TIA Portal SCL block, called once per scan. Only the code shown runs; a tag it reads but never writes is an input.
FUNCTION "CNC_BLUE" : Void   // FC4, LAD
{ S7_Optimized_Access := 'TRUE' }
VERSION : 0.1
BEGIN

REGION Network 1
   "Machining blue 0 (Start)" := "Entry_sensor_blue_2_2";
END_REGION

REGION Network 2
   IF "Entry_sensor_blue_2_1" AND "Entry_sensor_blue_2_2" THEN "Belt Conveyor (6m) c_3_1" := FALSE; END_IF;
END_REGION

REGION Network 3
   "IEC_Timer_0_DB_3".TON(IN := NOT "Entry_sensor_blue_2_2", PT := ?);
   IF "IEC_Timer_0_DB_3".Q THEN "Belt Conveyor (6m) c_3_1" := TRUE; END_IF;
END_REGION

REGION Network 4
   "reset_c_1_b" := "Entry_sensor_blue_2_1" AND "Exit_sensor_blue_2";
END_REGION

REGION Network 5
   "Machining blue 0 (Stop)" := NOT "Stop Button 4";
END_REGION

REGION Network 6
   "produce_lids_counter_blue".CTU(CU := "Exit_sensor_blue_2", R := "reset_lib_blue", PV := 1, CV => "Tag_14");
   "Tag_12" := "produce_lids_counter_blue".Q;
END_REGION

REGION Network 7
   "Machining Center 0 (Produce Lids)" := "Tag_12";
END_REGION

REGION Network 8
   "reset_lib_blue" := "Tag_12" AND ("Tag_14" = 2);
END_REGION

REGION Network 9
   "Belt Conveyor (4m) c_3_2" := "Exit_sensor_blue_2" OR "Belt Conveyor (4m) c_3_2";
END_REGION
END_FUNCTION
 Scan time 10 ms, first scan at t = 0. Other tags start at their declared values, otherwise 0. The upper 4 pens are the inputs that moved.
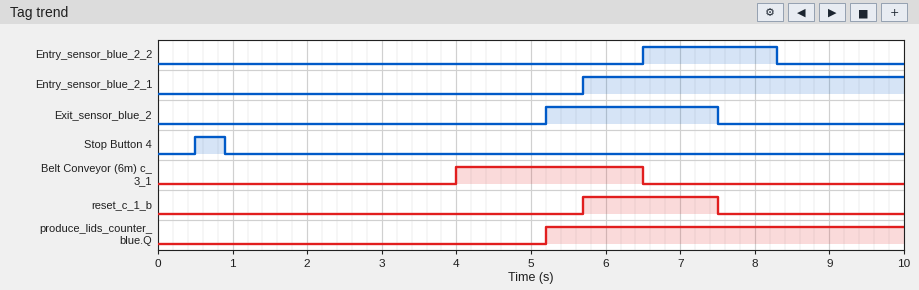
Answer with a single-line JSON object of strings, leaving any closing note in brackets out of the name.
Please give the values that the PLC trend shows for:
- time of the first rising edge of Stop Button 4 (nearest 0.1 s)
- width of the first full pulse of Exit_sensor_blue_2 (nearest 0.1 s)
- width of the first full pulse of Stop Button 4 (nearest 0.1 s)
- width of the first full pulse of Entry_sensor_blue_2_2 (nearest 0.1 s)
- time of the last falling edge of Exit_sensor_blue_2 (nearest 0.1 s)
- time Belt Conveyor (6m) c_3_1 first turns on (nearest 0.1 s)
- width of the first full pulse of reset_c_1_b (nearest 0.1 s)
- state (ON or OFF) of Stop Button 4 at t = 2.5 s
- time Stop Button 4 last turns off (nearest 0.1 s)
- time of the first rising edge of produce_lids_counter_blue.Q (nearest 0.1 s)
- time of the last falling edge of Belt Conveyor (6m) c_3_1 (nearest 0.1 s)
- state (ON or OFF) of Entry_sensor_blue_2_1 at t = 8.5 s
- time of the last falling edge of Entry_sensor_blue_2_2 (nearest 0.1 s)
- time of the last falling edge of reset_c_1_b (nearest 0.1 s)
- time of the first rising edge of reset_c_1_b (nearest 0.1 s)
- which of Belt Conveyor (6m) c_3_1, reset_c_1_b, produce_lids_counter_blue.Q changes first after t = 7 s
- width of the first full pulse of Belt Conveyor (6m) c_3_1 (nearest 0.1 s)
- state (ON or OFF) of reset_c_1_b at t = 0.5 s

{"time of the first rising edge of Stop Button 4": "0.5 s", "width of the first full pulse of Exit_sensor_blue_2": "2.3 s", "width of the first full pulse of Stop Button 4": "0.4 s", "width of the first full pulse of Entry_sensor_blue_2_2": "1.8 s", "time of the last falling edge of Exit_sensor_blue_2": "7.5 s", "time Belt Conveyor (6m) c_3_1 first turns on": "4.0 s", "width of the first full pulse of reset_c_1_b": "1.8 s", "state (ON or OFF) of Stop Button 4 at t = 2.5 s": "OFF", "time Stop Button 4 last turns off": "0.9 s", "time of the first rising edge of produce_lids_counter_blue.Q": "5.2 s", "time of the last falling edge of Belt Conveyor (6m) c_3_1": "6.5 s", "state (ON or OFF) of Entry_sensor_blue_2_1 at t = 8.5 s": "ON", "time of the last falling edge of Entry_sensor_blue_2_2": "8.3 s", "time of the last falling edge of reset_c_1_b": "7.5 s", "time of the first rising edge of reset_c_1_b": "5.7 s", "which of Belt Conveyor (6m) c_3_1, reset_c_1_b, produce_lids_counter_blue.Q changes first after t = 7 s": "reset_c_1_b", "width of the first full pulse of Belt Conveyor (6m) c_3_1": "2.5 s", "state (ON or OFF) of reset_c_1_b at t = 0.5 s": "OFF"}
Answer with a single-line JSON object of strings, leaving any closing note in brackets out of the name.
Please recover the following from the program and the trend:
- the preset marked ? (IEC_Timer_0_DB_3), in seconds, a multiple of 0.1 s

{"the preset marked ? (IEC_Timer_0_DB_3), in seconds, a multiple of 0.1 s": "4.0 s"}
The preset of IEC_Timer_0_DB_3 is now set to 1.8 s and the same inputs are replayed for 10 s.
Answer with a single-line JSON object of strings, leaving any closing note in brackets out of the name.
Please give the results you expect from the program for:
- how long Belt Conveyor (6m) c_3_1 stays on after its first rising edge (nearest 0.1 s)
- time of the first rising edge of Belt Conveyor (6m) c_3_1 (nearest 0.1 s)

{"how long Belt Conveyor (6m) c_3_1 stays on after its first rising edge": "4.7 s", "time of the first rising edge of Belt Conveyor (6m) c_3_1": "1.8 s"}
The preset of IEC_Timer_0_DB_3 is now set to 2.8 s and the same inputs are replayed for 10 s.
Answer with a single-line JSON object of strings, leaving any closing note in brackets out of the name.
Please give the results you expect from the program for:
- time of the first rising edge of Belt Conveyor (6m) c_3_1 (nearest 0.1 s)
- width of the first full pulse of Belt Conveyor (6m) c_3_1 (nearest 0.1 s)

{"time of the first rising edge of Belt Conveyor (6m) c_3_1": "2.8 s", "width of the first full pulse of Belt Conveyor (6m) c_3_1": "3.7 s"}
